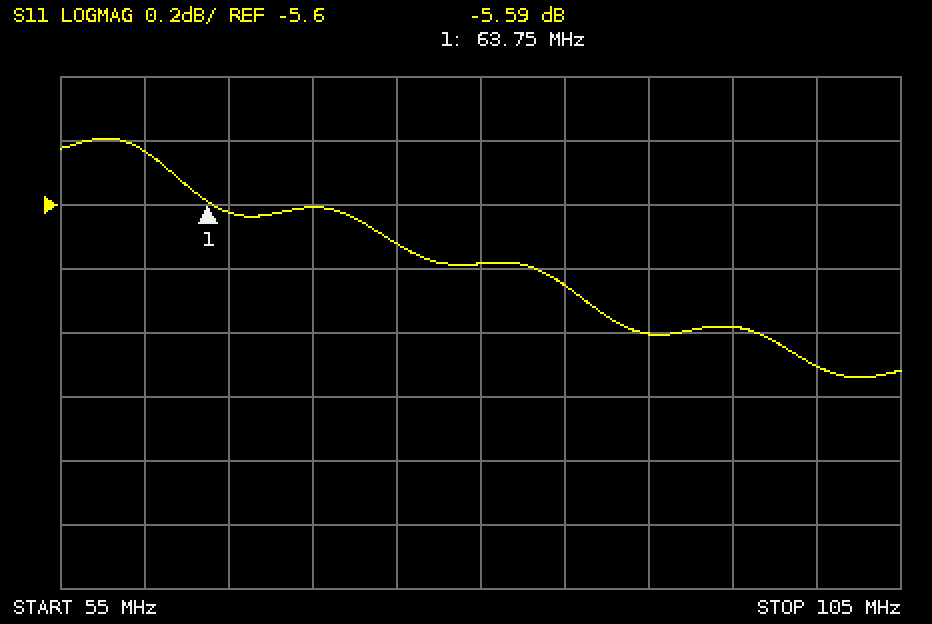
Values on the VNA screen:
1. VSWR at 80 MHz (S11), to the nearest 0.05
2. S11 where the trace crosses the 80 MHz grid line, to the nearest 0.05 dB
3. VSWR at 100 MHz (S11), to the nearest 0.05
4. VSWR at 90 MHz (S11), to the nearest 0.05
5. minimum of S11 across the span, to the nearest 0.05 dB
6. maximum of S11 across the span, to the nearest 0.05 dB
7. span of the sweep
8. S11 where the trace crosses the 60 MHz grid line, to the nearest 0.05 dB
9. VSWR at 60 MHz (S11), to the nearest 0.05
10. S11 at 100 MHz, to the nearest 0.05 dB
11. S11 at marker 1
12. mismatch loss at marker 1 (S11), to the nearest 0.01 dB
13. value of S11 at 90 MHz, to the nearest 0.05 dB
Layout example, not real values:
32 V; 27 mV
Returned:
3.10; -5.80 dB; 2.95; 3.00; -6.15 dB; -5.40 dB; 50 MHz; -5.45 dB; 3.30; -6.10 dB; -5.59 dB; 1.40 dB; -6.00 dB
